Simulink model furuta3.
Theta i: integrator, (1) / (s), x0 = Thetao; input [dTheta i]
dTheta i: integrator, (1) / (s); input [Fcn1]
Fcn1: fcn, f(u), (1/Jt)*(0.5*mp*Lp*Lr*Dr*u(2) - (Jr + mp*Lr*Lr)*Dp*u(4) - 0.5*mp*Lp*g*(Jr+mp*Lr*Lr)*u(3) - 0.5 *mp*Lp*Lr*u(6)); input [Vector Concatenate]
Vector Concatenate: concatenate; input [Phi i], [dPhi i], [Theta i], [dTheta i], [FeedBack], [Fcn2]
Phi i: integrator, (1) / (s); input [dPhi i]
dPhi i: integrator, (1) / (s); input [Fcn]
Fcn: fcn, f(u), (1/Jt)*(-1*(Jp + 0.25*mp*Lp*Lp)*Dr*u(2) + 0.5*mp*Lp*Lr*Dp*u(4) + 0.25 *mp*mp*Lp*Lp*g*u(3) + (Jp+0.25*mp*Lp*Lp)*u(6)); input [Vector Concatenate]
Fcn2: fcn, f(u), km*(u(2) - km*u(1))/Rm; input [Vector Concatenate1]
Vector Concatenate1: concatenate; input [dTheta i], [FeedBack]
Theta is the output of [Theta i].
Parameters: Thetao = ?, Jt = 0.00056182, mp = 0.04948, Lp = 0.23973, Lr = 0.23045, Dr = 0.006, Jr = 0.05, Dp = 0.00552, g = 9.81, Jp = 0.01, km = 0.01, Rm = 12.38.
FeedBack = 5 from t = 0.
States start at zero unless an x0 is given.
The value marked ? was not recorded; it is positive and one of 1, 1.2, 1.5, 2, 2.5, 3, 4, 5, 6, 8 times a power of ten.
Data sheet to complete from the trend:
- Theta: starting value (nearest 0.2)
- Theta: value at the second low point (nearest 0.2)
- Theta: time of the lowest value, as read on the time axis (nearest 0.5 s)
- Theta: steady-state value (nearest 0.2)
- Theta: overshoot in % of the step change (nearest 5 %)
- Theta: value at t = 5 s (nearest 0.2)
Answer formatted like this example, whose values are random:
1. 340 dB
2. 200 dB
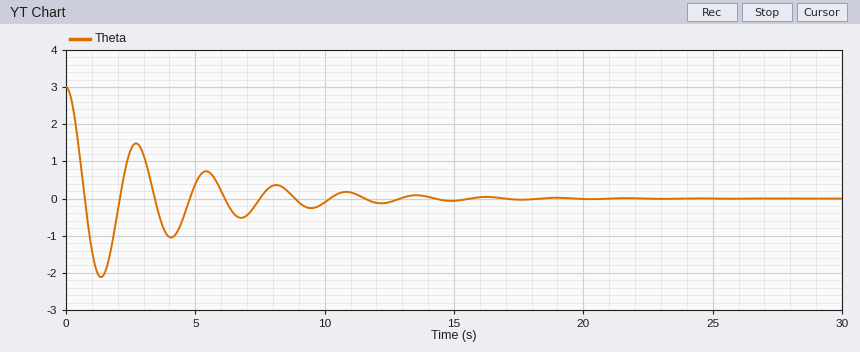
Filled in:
1. 3.0
2. -1.0
3. 1.5 s
4. 0.0
5. 70 %
6. 0.4
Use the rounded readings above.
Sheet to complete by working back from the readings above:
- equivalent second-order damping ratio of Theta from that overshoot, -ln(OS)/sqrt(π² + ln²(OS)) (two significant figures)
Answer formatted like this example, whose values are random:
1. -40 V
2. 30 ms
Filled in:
1. 0.11
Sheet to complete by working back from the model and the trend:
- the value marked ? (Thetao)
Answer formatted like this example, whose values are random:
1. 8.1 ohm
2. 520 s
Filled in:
1. 3
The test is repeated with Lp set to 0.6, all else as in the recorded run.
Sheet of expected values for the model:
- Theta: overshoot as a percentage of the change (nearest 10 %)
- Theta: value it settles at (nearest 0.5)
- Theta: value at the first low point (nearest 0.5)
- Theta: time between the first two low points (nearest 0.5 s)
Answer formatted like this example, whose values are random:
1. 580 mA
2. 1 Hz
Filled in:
1. 80 %
2. 0.0
3. -2.5
4. 1.5 s
